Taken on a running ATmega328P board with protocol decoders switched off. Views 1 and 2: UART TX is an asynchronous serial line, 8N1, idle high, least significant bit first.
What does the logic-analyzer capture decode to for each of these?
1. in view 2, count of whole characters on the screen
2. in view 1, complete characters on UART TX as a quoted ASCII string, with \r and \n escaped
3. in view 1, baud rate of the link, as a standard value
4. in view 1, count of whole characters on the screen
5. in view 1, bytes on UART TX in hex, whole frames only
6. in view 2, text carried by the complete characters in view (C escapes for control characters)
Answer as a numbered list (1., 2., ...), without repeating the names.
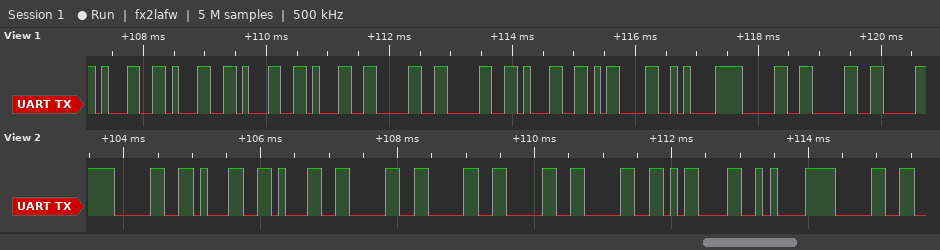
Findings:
1. 10
2. "1111001\r\n00"
3. 9600 baud
4. 11
5. 31 31 31 31 30 30 31 0D 0A 30 30
6. "0110000\r\n0"
